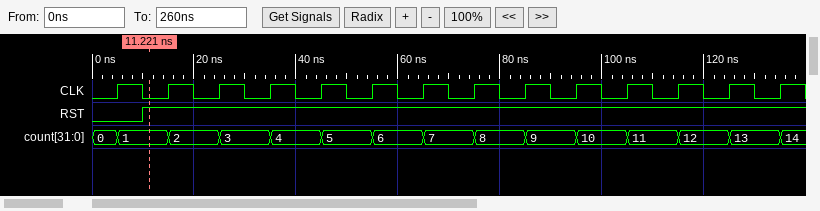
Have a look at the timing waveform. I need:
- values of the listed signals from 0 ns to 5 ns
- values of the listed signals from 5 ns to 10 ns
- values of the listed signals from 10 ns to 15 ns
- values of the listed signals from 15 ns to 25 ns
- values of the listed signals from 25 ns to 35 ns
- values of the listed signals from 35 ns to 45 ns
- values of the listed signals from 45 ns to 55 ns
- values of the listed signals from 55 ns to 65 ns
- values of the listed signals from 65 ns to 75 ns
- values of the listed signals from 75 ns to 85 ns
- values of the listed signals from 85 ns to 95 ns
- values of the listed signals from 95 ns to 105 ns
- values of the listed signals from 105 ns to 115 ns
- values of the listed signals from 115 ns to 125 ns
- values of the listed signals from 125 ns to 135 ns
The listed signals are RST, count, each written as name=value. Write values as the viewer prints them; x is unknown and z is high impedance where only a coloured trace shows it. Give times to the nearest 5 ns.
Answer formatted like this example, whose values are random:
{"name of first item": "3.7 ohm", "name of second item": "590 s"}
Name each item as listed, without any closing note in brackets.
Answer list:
{"values of the listed signals from 0 ns to 5 ns": "RST=0, count=0", "values of the listed signals from 5 ns to 10 ns": "RST=0, count=1", "values of the listed signals from 10 ns to 15 ns": "RST=1, count=1", "values of the listed signals from 15 ns to 25 ns": "RST=1, count=2", "values of the listed signals from 25 ns to 35 ns": "RST=1, count=3", "values of the listed signals from 35 ns to 45 ns": "RST=1, count=4", "values of the listed signals from 45 ns to 55 ns": "RST=1, count=5", "values of the listed signals from 55 ns to 65 ns": "RST=1, count=6", "values of the listed signals from 65 ns to 75 ns": "RST=1, count=7", "values of the listed signals from 75 ns to 85 ns": "RST=1, count=8", "values of the listed signals from 85 ns to 95 ns": "RST=1, count=9", "values of the listed signals from 95 ns to 105 ns": "RST=1, count=10", "values of the listed signals from 105 ns to 115 ns": "RST=1, count=11", "values of the listed signals from 115 ns to 125 ns": "RST=1, count=12", "values of the listed signals from 125 ns to 135 ns": "RST=1, count=13"}
